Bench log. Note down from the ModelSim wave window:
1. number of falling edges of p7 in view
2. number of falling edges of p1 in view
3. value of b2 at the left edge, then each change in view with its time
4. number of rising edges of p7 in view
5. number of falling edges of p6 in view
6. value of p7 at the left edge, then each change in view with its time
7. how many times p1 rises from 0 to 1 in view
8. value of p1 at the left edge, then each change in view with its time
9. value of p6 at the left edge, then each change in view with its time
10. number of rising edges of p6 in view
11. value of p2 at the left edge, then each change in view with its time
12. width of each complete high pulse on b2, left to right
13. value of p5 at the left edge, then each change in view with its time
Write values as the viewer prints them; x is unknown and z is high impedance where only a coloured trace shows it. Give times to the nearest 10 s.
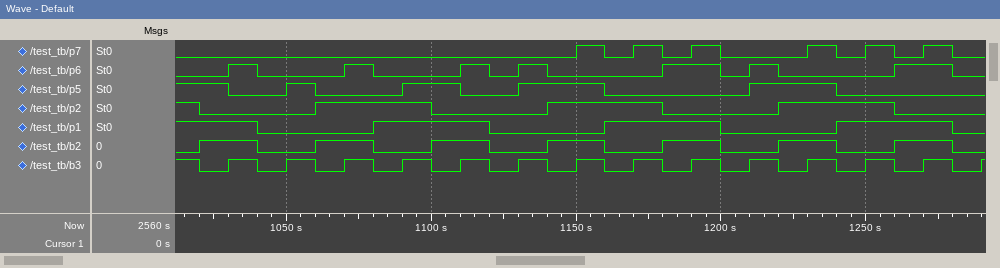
6
4
0, 1 at 1020 s, 0 at 1040 s, 1 at 1060 s, 0 at 1080 s, 1 at 1100 s, 0 at 1120 s, 1 at 1140 s, 0 at 1160 s, 1 at 1180 s, 0 at 1200 s, 1 at 1220 s, 0 at 1240 s, 1 at 1260 s, 0 at 1280 s
6
7
0, 1 at 1150 s, 0 at 1160 s, 1 at 1170 s, 0 at 1180 s, 1 at 1190 s, 0 at 1200 s, 1 at 1230 s, 0 at 1240 s, 1 at 1250 s, 0 at 1260 s, 1 at 1270 s, 0 at 1280 s
3
1, 0 at 1040 s, 1 at 1080 s, 0 at 1120 s, 1 at 1160 s, 0 at 1200 s, 1 at 1240 s, 0 at 1280 s
0, 1 at 1030 s, 0 at 1040 s, 1 at 1070 s, 0 at 1080 s, 1 at 1110 s, 0 at 1120 s, 1 at 1130 s, 0 at 1140 s, 1 at 1180 s, 0 at 1200 s, 1 at 1210 s, 0 at 1220 s, 1 at 1260 s, 0 at 1280 s
7
1, 0 at 1020 s, 1 at 1060 s, 0 at 1100 s, 1 at 1140 s, 0 at 1180 s, 1 at 1220 s, 0 at 1260 s
20 s, 20 s, 20 s, 20 s, 20 s, 20 s, 20 s
1, 0 at 1030 s, 1 at 1050 s, 0 at 1060 s, 1 at 1090 s, 0 at 1110 s, 1 at 1130 s, 0 at 1160 s, 1 at 1210 s, 0 at 1240 s
